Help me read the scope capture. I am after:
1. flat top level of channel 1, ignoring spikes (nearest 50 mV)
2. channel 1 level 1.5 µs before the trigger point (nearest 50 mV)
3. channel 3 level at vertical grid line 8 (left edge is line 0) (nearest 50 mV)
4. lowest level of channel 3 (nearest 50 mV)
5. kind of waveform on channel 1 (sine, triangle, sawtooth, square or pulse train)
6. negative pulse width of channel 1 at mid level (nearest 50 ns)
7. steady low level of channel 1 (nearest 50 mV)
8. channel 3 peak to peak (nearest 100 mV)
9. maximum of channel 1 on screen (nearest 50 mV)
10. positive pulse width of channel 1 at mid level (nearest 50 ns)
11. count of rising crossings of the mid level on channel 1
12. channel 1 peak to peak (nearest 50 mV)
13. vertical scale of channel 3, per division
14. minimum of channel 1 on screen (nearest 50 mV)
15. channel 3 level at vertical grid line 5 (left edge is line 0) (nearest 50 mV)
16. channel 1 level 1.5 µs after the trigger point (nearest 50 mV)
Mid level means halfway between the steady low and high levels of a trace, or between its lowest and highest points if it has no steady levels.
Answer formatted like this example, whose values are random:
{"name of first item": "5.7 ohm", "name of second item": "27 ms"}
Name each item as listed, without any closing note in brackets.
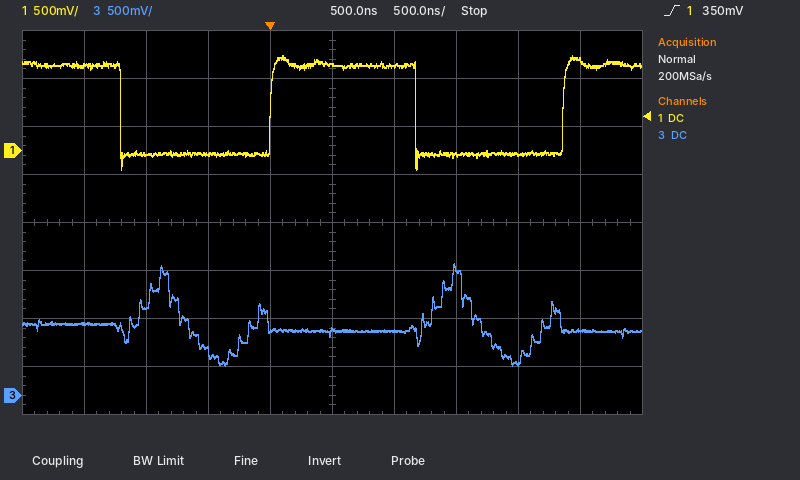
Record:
{"flat top level of channel 1, ignoring spikes": "900 mV", "channel 1 level 1.5 µs before the trigger point": "900 mV", "channel 3 level at vertical grid line 8 (left edge is line 0)": "350 mV", "lowest level of channel 3": "300 mV", "kind of waveform on channel 1": "square", "negative pulse width of channel 1 at mid level": "1.20 µs", "steady low level of channel 1": "-50 mV", "channel 3 peak to peak": "1.10 V", "maximum of channel 1 on screen": "1.00 V", "positive pulse width of channel 1 at mid level": "1.15 µs", "count of rising crossings of the mid level on channel 1": "2", "channel 1 peak to peak": "1.20 V", "vertical scale of channel 3, per division": "500 mV", "minimum of channel 1 on screen": "-200 mV", "channel 3 level at vertical grid line 5 (left edge is line 0)": "650 mV", "channel 1 level 1.5 µs after the trigger point": "-50 mV"}
